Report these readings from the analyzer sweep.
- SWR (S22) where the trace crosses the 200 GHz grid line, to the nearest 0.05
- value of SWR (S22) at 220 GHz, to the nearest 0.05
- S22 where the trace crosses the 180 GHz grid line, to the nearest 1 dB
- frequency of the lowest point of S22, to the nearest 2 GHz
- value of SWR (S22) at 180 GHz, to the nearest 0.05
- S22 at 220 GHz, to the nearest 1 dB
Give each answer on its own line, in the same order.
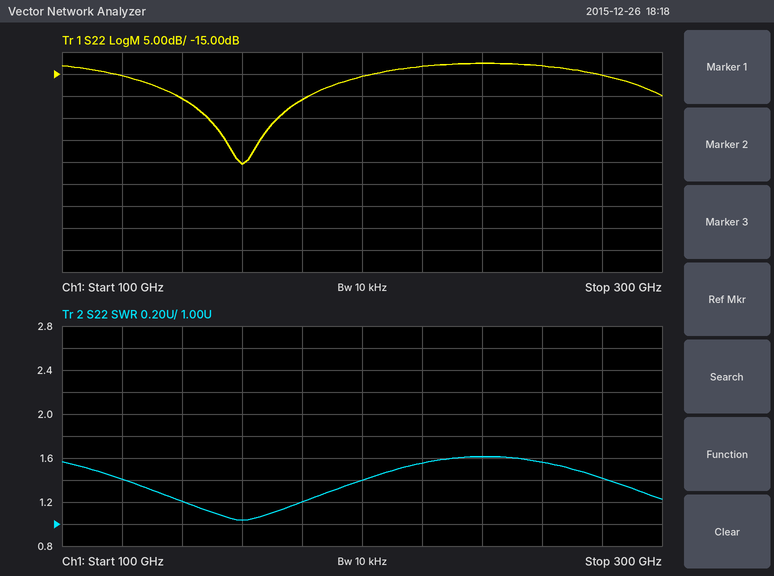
1.40
1.55
-21 dB
160 GHz
1.20
-13 dB
